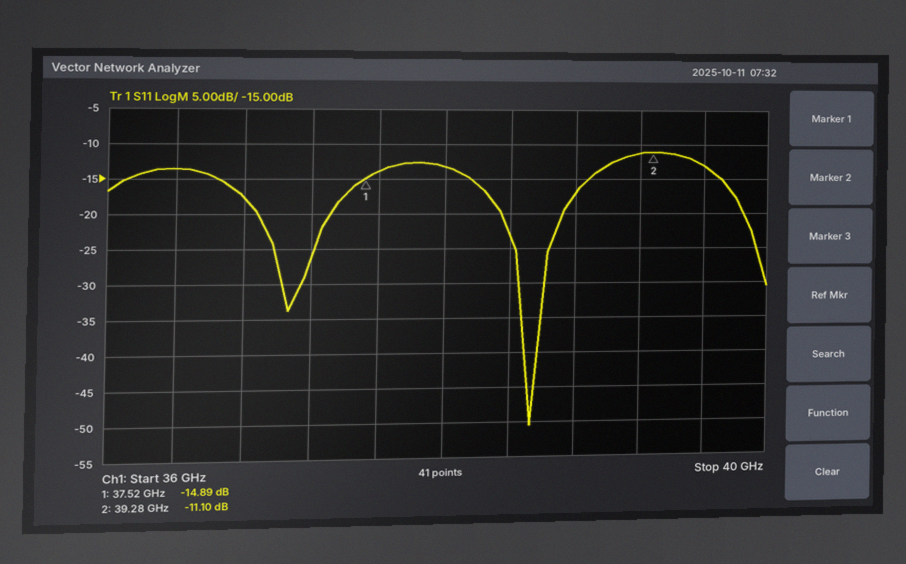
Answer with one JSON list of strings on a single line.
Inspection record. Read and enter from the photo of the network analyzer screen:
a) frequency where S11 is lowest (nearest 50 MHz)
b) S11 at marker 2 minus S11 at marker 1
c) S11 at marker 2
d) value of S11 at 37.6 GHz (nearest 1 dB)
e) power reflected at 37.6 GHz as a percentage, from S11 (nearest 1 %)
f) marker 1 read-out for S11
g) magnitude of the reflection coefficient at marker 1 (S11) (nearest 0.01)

["38.55 GHz", "3.79 dB", "-11.10 dB", "-14 dB", "4 %", "-14.89 dB", "0.18"]
